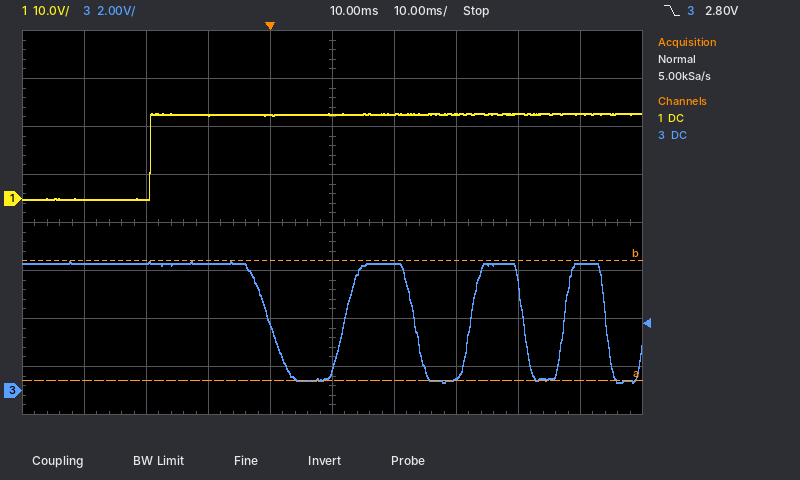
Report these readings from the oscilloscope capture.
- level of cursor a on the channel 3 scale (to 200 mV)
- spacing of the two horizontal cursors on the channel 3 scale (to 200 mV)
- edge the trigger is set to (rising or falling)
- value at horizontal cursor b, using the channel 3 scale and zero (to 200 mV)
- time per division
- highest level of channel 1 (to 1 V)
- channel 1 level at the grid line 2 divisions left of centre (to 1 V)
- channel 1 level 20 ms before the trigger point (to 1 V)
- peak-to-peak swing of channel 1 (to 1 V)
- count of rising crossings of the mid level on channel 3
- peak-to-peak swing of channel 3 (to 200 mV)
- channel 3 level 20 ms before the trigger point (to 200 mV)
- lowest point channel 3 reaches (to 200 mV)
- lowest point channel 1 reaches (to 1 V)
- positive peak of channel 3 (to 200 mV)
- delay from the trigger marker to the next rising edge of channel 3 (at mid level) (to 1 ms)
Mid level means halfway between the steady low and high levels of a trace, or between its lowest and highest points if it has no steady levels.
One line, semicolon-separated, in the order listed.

400 mV; 5.0 V; falling; 5.4 V; 10 ms; 18 V; 17 V; 0 V; 18 V; 3; 5.0 V; 5.4 V; 400 mV; 0 V; 5.4 V; 12 ms
